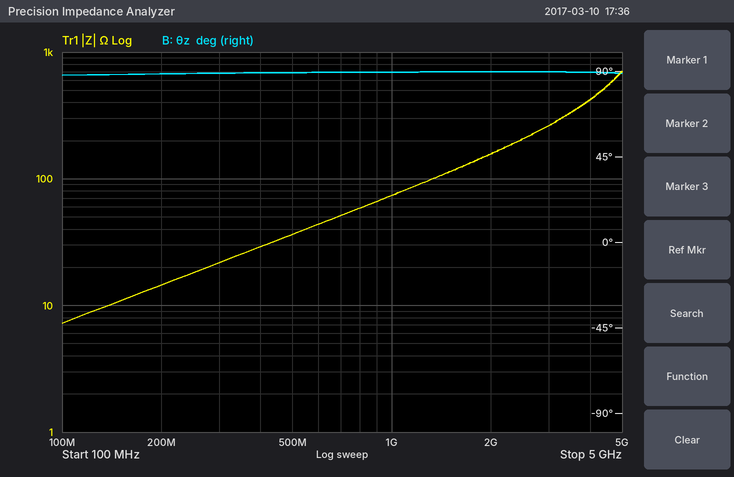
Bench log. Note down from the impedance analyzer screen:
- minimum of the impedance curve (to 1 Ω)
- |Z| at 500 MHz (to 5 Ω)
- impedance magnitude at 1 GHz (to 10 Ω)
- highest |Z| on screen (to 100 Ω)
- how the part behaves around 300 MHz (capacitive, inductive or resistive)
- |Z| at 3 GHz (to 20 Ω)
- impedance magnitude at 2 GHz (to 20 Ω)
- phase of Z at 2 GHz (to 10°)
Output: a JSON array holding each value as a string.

["7 Ω", "35 Ω", "70 Ω", "700 Ω", "inductive", "260 Ω", "160 Ω", "90°"]
